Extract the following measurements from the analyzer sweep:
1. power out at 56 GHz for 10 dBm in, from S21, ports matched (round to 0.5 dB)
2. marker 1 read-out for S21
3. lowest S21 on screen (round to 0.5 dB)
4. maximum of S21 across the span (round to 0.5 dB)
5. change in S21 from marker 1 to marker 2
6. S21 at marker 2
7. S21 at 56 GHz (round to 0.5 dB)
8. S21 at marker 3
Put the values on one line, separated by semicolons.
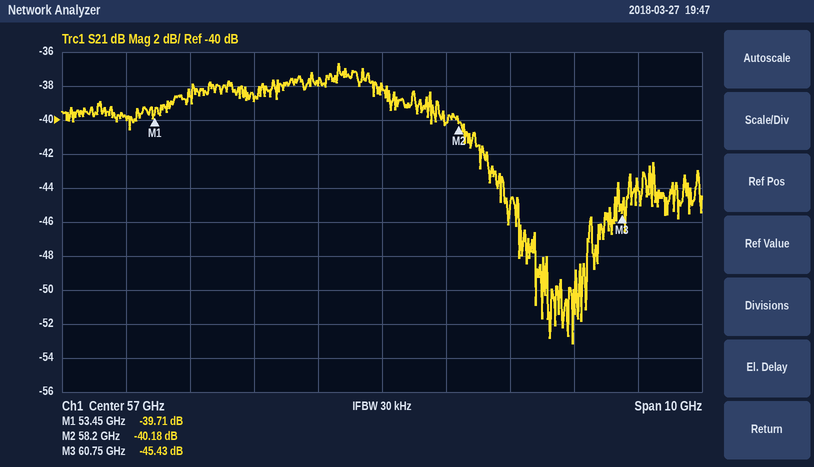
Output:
-28.0 dBm; -39.71 dB; -53.0 dB; -36.5 dB; -0.47 dB; -40.18 dB; -38.0 dB; -45.43 dB
